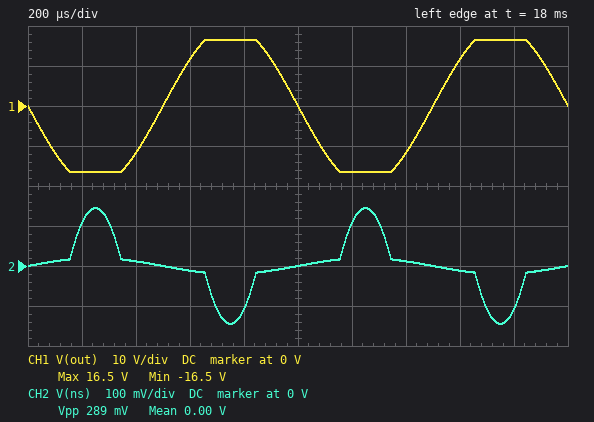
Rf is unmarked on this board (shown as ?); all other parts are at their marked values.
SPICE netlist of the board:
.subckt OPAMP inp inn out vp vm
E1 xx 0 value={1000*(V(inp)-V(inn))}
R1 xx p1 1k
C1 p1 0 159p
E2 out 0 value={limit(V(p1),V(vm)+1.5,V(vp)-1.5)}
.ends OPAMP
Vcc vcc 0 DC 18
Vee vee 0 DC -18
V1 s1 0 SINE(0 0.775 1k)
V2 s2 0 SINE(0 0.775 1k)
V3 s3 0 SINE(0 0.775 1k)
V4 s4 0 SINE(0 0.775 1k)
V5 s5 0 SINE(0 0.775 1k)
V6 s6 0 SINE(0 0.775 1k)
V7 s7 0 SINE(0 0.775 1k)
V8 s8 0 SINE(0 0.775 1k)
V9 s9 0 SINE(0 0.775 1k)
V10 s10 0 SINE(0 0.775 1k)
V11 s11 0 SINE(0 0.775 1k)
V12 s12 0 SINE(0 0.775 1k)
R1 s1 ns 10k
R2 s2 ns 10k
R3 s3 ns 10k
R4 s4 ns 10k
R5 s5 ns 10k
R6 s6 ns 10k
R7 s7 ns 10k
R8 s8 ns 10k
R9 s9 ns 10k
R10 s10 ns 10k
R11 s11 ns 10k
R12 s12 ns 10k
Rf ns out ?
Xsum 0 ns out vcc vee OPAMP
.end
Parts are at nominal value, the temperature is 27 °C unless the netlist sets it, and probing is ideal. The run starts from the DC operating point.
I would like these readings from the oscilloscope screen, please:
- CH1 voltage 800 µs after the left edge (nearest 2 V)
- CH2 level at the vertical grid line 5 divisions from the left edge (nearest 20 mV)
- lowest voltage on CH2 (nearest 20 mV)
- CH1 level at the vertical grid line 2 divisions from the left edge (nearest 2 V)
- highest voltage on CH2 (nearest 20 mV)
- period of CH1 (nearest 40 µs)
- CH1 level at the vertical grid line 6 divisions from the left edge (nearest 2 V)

16 V
0 V
-140 mV
-12 V
140 mV
1.00 ms
-16 V
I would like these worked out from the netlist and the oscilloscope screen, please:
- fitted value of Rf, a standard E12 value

22 kΩ
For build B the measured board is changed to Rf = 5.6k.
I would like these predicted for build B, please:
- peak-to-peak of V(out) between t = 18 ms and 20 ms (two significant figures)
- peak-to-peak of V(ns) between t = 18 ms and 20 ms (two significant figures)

10 V
10 mV
